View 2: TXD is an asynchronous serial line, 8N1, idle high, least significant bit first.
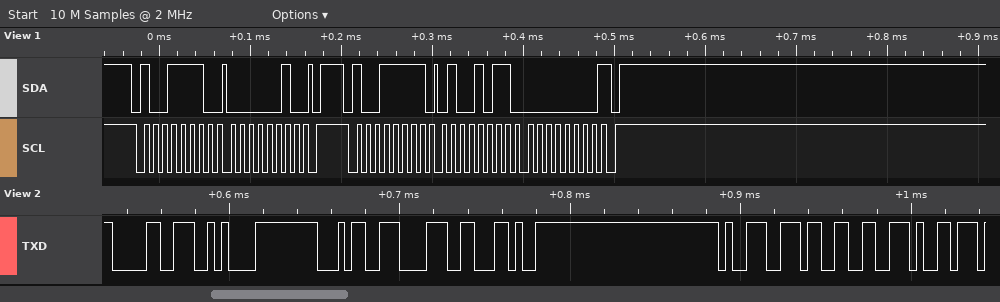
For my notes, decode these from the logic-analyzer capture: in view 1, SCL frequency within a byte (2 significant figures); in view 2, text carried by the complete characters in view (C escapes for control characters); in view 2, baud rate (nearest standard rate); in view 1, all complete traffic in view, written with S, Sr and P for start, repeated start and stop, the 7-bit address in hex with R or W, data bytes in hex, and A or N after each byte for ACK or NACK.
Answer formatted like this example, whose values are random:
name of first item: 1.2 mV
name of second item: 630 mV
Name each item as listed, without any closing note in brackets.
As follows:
in view 1, SCL frequency within a byte: 100 kHz
in view 2, text carried by the complete characters in view: "0\n48,93."
in view 2, baud rate: 250000 baud
in view 1, all complete traffic in view, written with S, Sr and P for start, repeated start and stop, the 7-bit address in hex with R or W, data bytes in hex, and A or N after each byte for ACK or NACK: S 4FW A 02 A P S 4FR A 4B A 00 N P
